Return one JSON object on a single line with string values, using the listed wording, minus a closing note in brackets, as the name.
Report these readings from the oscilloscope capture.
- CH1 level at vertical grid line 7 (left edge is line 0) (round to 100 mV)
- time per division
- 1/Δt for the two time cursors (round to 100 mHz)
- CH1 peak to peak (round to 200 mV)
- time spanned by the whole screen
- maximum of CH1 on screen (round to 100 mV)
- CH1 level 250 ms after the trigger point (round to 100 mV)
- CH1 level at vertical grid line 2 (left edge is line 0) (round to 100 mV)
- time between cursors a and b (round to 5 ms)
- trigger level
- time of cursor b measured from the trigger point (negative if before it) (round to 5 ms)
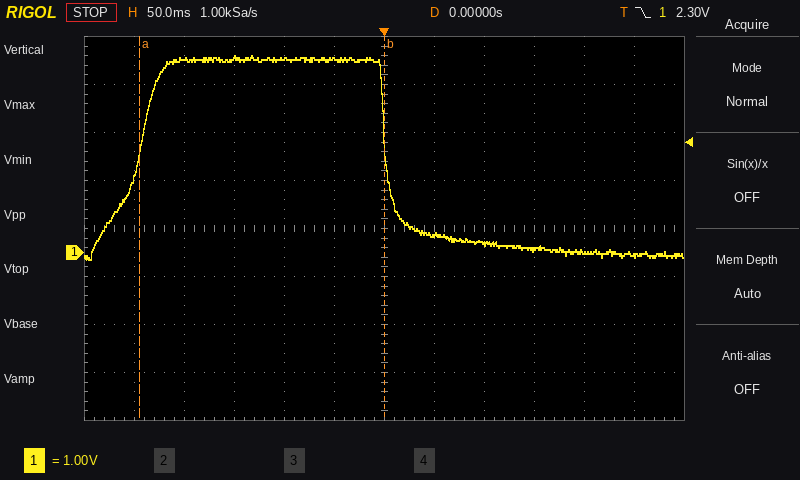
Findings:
{"CH1 level at vertical grid line 7 (left edge is line 0)": "400 mV", "time per division": "50 ms", "1/Δt for the two time cursors": "4.1 Hz", "CH1 peak to peak": "4.2 V", "time spanned by the whole screen": "600 ms", "maximum of CH1 on screen": "4.1 V", "CH1 level 250 ms after the trigger point": "-100 mV", "CH1 level at vertical grid line 2 (left edge is line 0)": "4.0 V", "time between cursors a and b": "245 ms", "trigger level": "2.30 V", "time of cursor b measured from the trigger point (negative if before it)": "0 ms"}
